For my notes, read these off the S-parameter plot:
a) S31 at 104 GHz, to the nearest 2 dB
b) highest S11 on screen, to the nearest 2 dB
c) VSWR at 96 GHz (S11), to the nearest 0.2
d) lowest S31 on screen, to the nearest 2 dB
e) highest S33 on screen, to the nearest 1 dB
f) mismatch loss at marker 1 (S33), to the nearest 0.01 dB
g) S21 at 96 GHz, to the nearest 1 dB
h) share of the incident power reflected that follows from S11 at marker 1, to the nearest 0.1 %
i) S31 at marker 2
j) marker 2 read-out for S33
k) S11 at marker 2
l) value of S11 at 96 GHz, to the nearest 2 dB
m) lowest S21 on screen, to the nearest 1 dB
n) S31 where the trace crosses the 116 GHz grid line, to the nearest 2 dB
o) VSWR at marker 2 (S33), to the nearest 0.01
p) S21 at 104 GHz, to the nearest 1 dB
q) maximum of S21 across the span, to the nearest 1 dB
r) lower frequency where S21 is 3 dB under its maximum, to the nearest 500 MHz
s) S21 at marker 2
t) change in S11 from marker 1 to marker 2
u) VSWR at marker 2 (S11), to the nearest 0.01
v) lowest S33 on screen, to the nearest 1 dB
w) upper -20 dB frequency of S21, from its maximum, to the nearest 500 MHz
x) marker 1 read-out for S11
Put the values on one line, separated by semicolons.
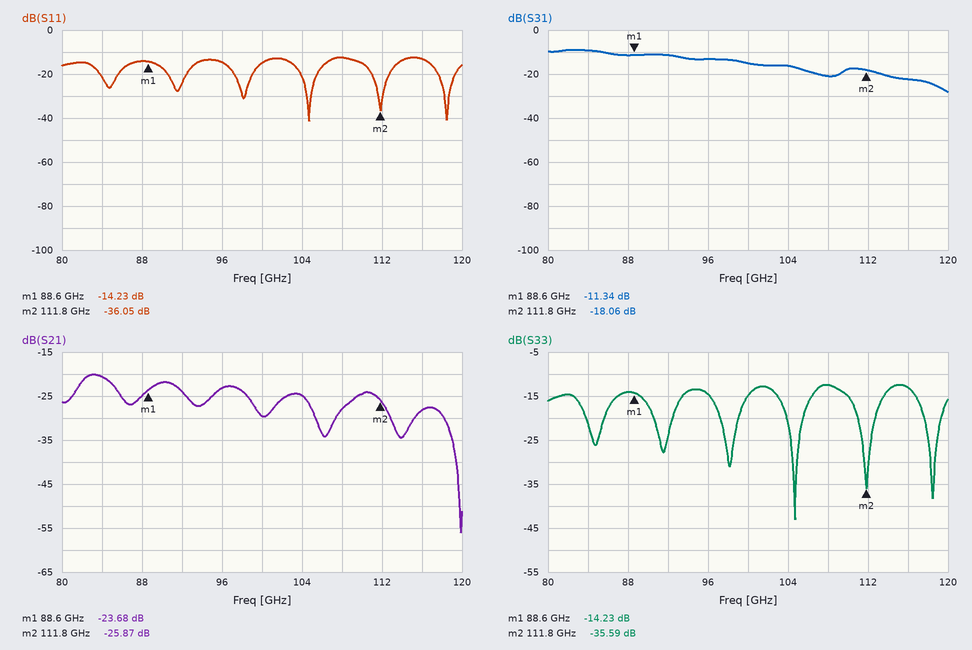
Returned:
-16 dB; -12 dB; 1.4; -28 dB; -12 dB; 0.17 dB; -23 dB; 3.8 %; -18.06 dB; -35.59 dB; -36.05 dB; -14 dB; -56 dB; -22 dB; 1.03; -25 dB; -20 dB; 81.5 GHz; -25.87 dB; -21.82 dB; 1.03; -43 dB; 119.5 GHz; -14.23 dB
